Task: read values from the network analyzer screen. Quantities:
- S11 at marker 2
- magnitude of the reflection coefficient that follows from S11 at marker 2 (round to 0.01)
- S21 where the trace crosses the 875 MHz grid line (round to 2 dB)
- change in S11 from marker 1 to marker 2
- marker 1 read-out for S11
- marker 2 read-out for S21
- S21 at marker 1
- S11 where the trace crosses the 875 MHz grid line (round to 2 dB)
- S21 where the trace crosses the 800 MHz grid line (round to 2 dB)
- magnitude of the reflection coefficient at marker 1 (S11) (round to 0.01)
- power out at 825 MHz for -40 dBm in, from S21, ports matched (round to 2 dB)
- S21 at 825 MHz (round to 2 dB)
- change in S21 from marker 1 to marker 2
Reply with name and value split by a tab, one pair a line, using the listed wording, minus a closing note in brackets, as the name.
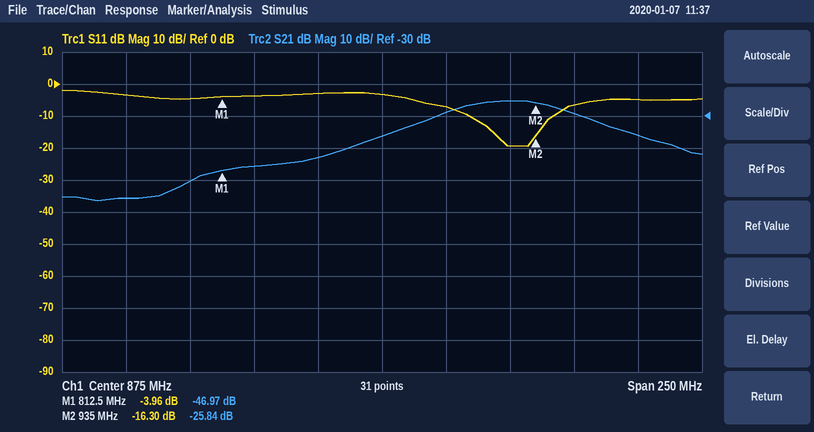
S11 at marker 2	-16.30 dB
magnitude of the reflection coefficient that follows from S11 at marker 2	0.15
S21 where the trace crosses the 875 MHz grid line	-36 dB
change in S11 from marker 1 to marker 2	-12.34 dB
marker 1 read-out for S11	-3.96 dB
marker 2 read-out for S21	-25.84 dB
S21 at marker 1	-46.97 dB
S11 where the trace crosses the 875 MHz grid line	-4 dB
S21 where the trace crosses the 800 MHz grid line	-50 dB
magnitude of the reflection coefficient at marker 1 (S11)	0.63
power out at 825 MHz for -40 dBm in, from S21, ports matched	-86 dBm
S21 at 825 MHz	-46 dB
change in S21 from marker 1 to marker 2	21.13 dB
